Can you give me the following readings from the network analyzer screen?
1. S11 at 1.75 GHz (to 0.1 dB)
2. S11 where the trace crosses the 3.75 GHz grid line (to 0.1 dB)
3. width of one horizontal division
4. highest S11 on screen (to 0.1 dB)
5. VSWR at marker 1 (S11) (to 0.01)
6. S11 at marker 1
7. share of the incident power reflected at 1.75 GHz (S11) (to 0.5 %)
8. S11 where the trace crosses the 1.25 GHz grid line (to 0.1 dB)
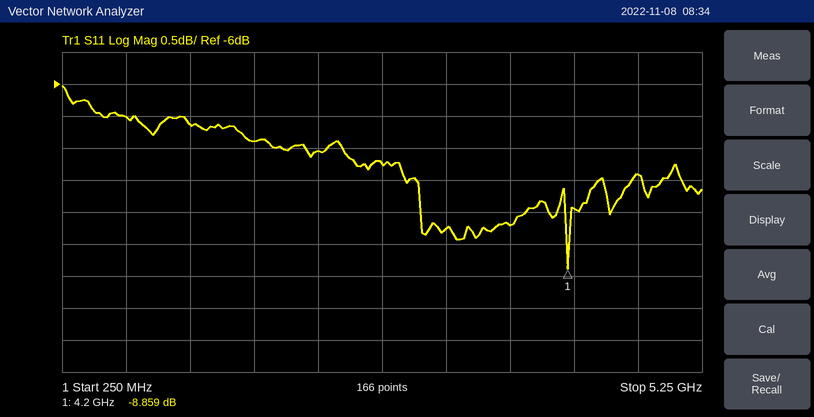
-6.9 dB
-8.2 dB
500 MHz
-6.0 dB
2.13
-8.859 dB
20.5 %
-6.6 dB
